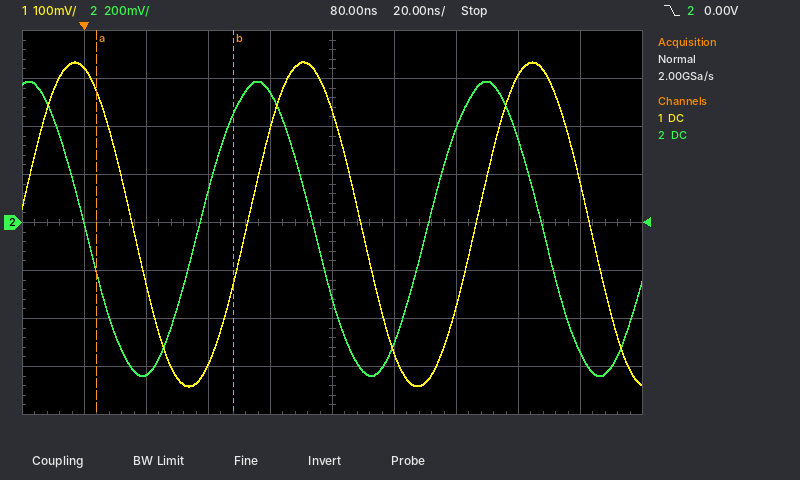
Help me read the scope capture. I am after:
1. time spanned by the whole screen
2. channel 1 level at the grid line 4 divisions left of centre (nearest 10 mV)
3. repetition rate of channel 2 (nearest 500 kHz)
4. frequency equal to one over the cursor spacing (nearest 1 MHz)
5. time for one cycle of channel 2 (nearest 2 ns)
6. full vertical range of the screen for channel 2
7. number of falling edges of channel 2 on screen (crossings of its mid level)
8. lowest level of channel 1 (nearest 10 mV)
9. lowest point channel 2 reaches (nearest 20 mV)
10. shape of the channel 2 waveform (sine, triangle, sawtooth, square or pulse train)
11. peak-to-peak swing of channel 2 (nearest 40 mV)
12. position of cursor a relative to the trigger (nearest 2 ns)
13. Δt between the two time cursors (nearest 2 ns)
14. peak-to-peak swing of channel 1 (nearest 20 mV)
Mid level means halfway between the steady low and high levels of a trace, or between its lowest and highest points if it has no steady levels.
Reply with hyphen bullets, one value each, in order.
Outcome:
- 200 ns
- 320 mV
- 13.5 MHz
- 23 MHz
- 74 ns
- 1.6 V
- 3
- -340 mV
- -640 mV
- sine
- 1.24 V
- +4 ns
- 44 ns
- 680 mV
